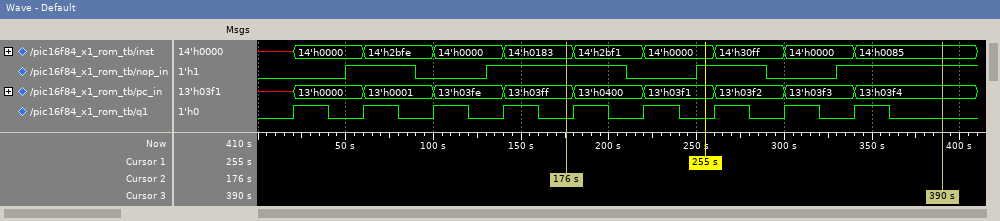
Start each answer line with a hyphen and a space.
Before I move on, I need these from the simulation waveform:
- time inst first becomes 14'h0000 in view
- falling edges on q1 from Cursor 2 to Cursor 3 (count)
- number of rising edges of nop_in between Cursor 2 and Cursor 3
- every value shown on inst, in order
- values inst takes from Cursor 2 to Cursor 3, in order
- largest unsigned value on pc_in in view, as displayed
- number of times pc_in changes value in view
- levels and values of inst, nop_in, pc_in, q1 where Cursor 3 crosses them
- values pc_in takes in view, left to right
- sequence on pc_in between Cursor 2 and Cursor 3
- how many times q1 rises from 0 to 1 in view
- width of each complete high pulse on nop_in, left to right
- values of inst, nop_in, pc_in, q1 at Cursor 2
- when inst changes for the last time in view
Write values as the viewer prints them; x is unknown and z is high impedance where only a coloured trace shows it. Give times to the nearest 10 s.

- 20 s
- 5
- 2
- x, 14'h0000, 14'h2bfe, 14'h0000, 14'h0183, 14'h2bf1, 14'h0000, 14'h30ff, 14'h0000, 14'h0085
- 14'h0183, 14'h2bf1, 14'h0000, 14'h30ff, 14'h0000, 14'h0085
- 13'h0400
- 9
- inst=14'h0085, nop_in=1, pc_in=13'h03f4, q1=0
- x, 13'h0000, 13'h0001, 13'h03fe, 13'h03ff, 13'h0400, 13'h03f1, 13'h03f2, 13'h03f3, 13'h03f4
- 13'h03ff, 13'h0400, 13'h03f1, 13'h03f2, 13'h03f3, 13'h03f4
- 9
- 40 s, 80 s, 40 s
- inst=14'h0183, nop_in=1, pc_in=13'h03ff, q1=0
- 340 s
